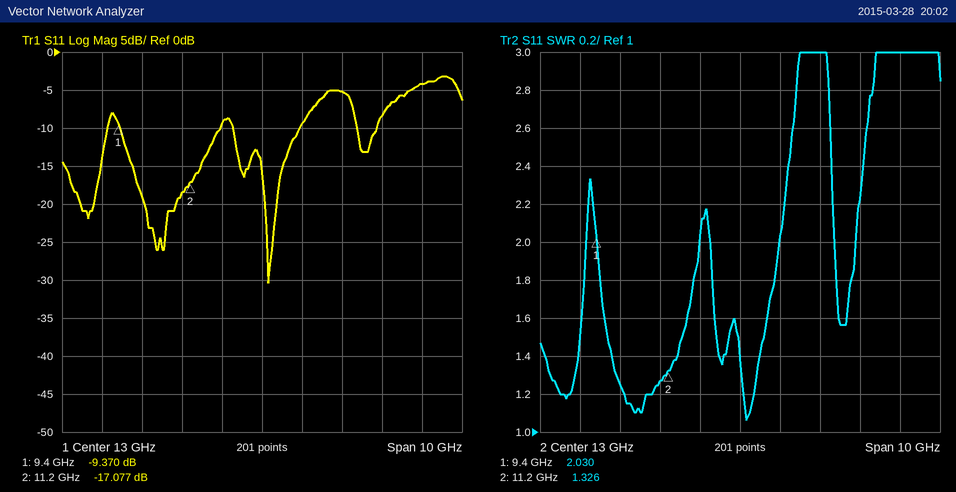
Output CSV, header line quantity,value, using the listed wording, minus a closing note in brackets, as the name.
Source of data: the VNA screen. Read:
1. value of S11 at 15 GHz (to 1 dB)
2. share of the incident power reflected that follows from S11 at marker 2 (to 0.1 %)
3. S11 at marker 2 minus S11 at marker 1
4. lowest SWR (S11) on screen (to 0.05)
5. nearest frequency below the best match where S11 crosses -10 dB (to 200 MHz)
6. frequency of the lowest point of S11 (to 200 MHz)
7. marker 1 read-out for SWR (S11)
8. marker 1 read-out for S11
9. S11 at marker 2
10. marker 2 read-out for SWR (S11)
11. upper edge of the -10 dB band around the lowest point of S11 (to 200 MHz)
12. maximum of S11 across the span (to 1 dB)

quantity,value
value of S11 at 15 GHz,-5 dB
share of the incident power reflected that follows from S11 at marker 2,2.0 %
S11 at marker 2 minus S11 at marker 1,-7.707 dB
lowest SWR (S11) on screen,1.05
nearest frequency below the best match where S11 crosses -10 dB,12.2 GHz
frequency of the lowest point of S11,13.2 GHz
marker 1 read-out for SWR,2.030
marker 1 read-out for S11,-9.370 dB
S11 at marker 2,-17.077 dB
marker 2 read-out for SWR,1.326
upper edge of the -10 dB band around the lowest point of S11,14.0 GHz
maximum of S11 across the span,-3 dB
